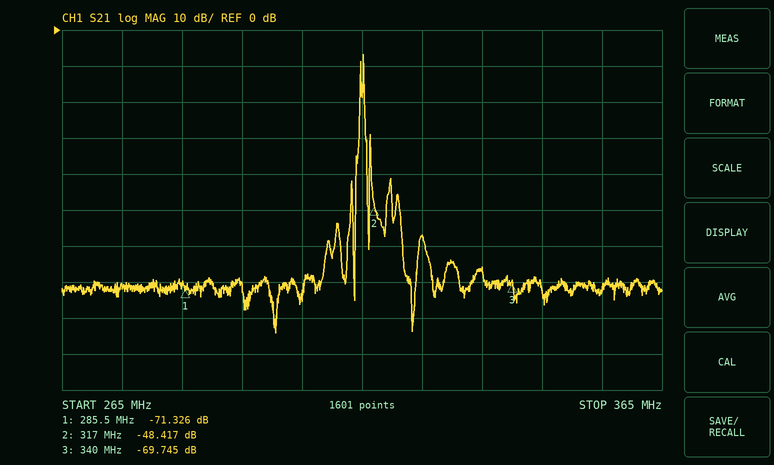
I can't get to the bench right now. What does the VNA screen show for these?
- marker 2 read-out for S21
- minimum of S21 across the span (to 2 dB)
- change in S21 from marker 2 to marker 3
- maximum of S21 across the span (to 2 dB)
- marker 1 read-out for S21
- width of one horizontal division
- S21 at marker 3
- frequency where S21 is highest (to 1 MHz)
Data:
-48.417 dB
-84 dB
-21.328 dB
-6 dB
-71.326 dB
10 MHz
-69.745 dB
315 MHz
